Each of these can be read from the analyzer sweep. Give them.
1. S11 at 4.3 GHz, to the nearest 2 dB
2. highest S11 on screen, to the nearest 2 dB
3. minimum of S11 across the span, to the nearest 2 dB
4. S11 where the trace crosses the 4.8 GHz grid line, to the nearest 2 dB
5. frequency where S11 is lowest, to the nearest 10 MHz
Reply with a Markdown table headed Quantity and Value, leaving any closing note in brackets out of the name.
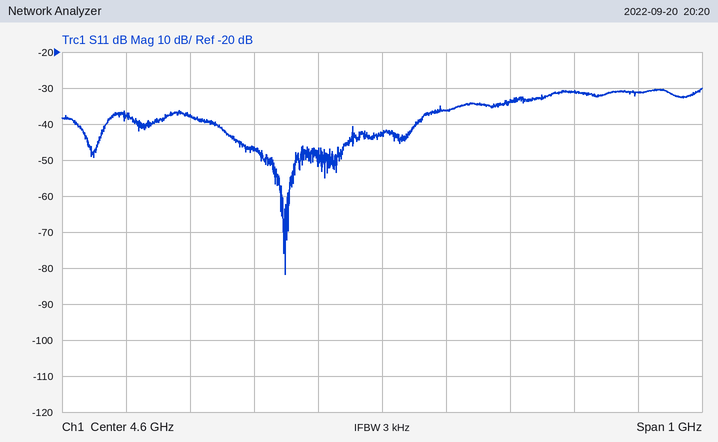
| Quantity | Value |
|---|---|
| S11 at 4.3 GHz, to the nearest 2 dB | -38 dB |
| highest S11 on screen, to the nearest 2 dB | -30 dB |
| minimum of S11 across the span, to the nearest 2 dB | -82 dB |
| S11 where the trace crosses the 4.8 GHz grid line, to the nearest 2 dB | -34 dB |
| frequency where S11 is lowest, to the nearest 10 MHz | 4.45 GHz |
